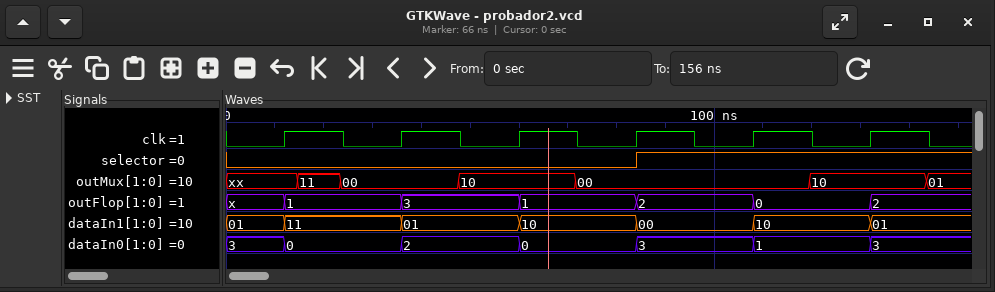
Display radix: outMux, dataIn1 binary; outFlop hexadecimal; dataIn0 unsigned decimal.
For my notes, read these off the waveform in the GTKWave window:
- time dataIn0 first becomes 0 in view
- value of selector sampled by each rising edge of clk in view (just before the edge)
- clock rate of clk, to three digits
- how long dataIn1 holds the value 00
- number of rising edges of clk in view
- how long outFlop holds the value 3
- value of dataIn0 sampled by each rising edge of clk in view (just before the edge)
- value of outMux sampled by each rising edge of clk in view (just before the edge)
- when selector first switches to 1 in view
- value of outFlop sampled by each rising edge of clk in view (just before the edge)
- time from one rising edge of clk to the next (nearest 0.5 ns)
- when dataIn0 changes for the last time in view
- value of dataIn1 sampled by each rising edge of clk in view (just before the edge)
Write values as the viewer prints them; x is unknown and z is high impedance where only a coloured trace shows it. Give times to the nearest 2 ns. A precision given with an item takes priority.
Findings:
12 ns
0 0 0 0 1 1
41.7 MHz
24 ns
6
24 ns
3, 0, 2, 0, 3, 1
xx, 00, 10, 00, 00, 10
84 ns
x, 1, 3, 1, 2, 0
24 ns
132 ns
01, 11, 01, 10, 00, 10
